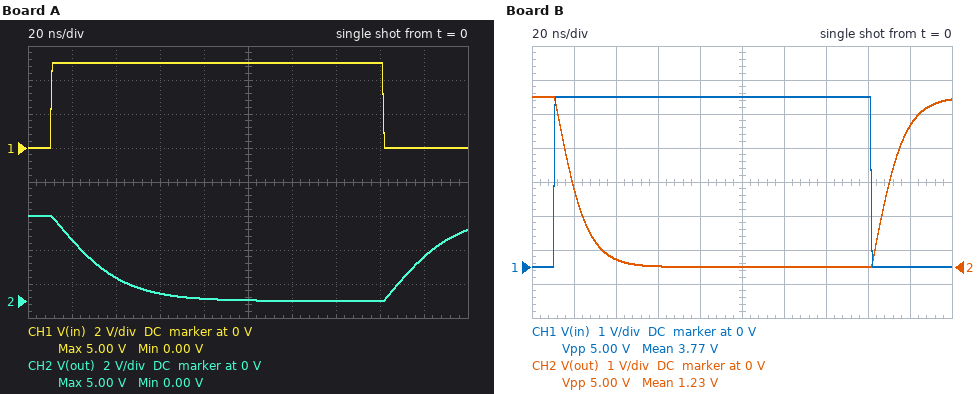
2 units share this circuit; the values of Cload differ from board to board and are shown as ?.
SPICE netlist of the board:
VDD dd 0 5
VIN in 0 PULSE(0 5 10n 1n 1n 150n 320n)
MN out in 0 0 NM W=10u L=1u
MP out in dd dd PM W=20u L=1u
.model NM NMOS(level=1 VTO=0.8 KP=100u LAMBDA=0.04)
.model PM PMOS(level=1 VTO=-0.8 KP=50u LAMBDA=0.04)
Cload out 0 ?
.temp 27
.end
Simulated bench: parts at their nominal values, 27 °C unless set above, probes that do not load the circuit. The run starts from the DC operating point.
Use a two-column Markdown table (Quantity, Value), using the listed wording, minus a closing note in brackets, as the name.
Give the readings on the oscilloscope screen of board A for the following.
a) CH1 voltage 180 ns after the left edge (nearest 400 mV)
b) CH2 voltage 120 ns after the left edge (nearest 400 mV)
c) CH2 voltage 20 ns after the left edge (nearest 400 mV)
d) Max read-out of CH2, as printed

| Quantity | Value |
|---|---|
| CH1 voltage 180 ns after the left edge | 0 V |
| CH2 voltage 120 ns after the left edge | 0 V |
| CH2 voltage 20 ns after the left edge | 3.6 V |
| Max read-out of CH2, as printed | 5.00 V |
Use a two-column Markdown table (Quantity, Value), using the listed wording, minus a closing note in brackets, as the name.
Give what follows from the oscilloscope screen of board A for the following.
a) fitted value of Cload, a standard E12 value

| Quantity | Value |
|---|---|
| fitted value of Cload, a standard E12 value | 68 pF |
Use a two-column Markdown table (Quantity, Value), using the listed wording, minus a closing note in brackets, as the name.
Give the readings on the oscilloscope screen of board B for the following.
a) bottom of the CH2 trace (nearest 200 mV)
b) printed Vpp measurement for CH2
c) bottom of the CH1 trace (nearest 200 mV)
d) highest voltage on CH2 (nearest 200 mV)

| Quantity | Value |
|---|---|
| bottom of the CH2 trace | 0 V |
| printed Vpp measurement for CH2 | 5.00 V |
| bottom of the CH1 trace | 0 V |
| highest voltage on CH2 | 5.0 V |
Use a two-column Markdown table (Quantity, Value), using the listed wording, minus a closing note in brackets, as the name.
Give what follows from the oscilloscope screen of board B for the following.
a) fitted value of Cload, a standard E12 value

| Quantity | Value |
|---|---|
| fitted value of Cload, a standard E12 value | 33 pF |
